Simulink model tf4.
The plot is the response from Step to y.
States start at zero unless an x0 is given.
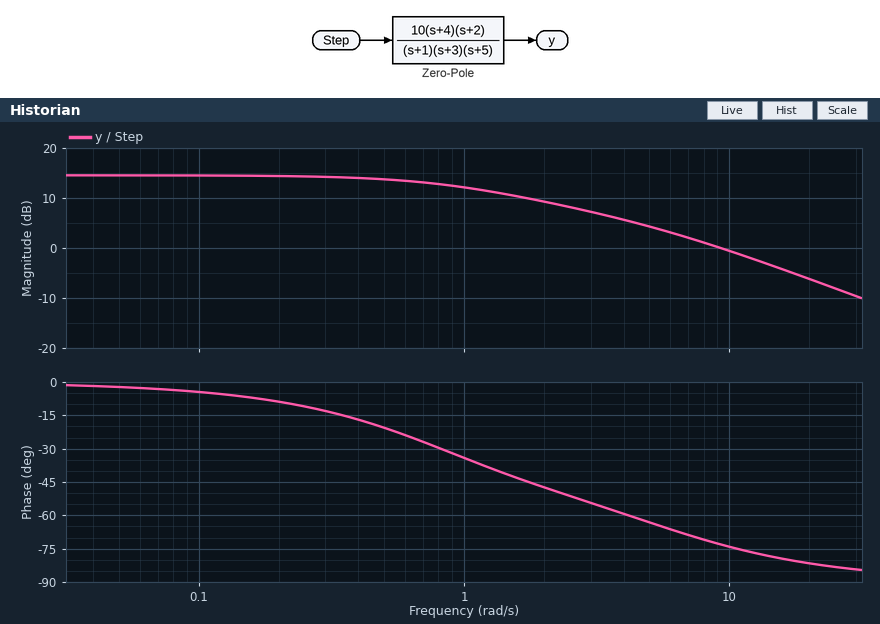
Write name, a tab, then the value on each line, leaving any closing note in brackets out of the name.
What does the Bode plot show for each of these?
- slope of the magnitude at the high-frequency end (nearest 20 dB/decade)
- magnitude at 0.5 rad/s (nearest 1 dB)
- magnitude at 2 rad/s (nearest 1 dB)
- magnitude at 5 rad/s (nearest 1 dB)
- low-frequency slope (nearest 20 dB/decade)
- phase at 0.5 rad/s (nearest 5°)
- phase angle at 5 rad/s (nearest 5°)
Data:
slope of the magnitude at the high-frequency end	-20 dB/decade
magnitude at 0.5 rad/s	14 dB
magnitude at 2 rad/s	9 dB
magnitude at 5 rad/s	4 dB
low-frequency slope	0 dB/decade
phase at 0.5 rad/s	-20°
phase angle at 5 rad/s	-65°
